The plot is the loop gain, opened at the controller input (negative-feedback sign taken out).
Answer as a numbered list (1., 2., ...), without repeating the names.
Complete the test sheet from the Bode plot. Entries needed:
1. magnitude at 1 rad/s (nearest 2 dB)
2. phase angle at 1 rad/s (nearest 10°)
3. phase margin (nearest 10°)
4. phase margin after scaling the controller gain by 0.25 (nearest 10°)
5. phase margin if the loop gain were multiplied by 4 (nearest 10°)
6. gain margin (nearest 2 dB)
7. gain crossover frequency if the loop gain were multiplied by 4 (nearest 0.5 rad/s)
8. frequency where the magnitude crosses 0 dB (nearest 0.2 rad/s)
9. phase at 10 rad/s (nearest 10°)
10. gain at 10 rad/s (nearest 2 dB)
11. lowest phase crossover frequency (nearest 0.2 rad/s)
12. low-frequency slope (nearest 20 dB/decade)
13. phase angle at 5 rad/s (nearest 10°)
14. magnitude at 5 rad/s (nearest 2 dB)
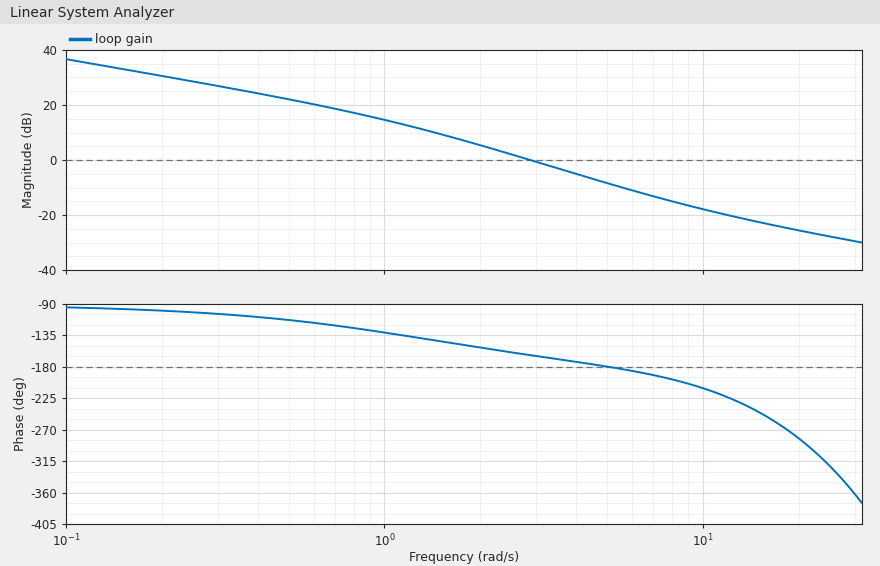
1. 14 dB
2. -130°
3. 20°
4. 40°
5. -10°
6. 8 dB
7. 6.5 rad/s
8. 2.8 rad/s
9. -210°
10. -18 dB
11. 5.0 rad/s
12. -20 dB/decade
13. -180°
14. -8 dB
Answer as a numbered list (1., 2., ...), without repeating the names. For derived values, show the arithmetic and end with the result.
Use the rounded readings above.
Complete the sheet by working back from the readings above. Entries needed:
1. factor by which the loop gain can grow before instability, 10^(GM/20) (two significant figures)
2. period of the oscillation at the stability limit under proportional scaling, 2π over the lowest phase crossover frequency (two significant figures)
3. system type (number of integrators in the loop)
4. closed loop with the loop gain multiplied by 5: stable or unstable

1. 10^(8 / 20) = 2.5
2. 2π / 5 = 1.3 s
3. 1
4. unstable
